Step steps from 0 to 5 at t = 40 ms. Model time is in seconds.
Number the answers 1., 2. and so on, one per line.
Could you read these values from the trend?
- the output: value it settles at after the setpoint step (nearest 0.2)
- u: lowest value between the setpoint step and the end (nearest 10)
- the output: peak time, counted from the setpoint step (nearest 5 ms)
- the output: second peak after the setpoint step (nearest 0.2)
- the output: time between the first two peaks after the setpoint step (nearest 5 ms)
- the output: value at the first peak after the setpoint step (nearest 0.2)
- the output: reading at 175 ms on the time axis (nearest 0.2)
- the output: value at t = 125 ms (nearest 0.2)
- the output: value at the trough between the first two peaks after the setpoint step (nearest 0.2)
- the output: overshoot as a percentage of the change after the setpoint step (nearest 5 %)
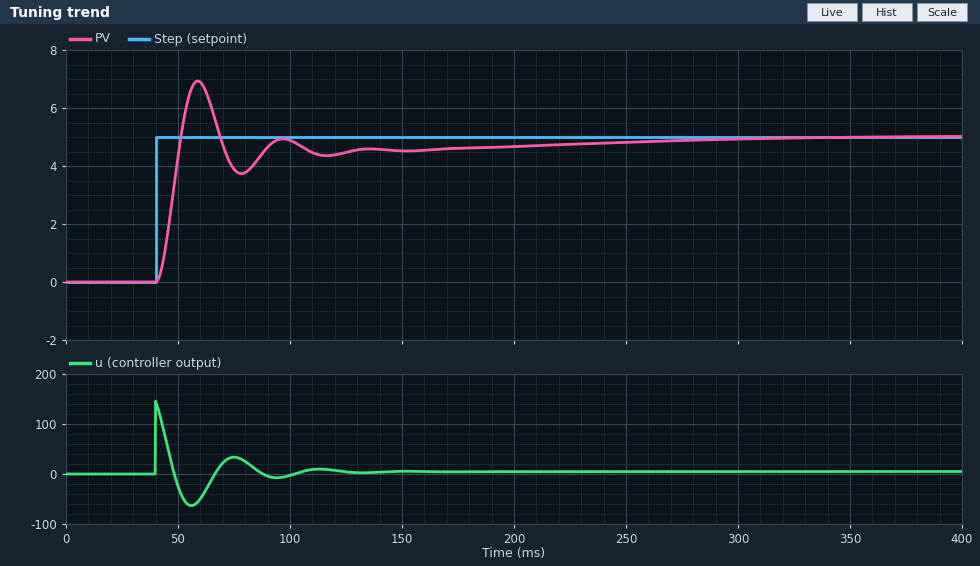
1. 5.0
2. -60
3. 20 ms
4. 5.0
5. 40 ms
6. 7.0
7. 4.6
8. 4.4
9. 3.8
10. 40 %
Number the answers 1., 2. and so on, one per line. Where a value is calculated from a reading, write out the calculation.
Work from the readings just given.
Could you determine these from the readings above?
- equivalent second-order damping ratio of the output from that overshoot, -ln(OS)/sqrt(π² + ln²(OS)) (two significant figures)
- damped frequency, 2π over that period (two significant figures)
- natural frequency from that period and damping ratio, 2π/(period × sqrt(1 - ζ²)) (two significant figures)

1. ln(0.4) = -0.916; 0.916 / sqrt(9.870 + 0.840) = 0.28
2. 2π / 40 = 0.16 rad/ms
3. 2π / (40 × sqrt(1 - 0.28²)) = 0.16 rad/ms
